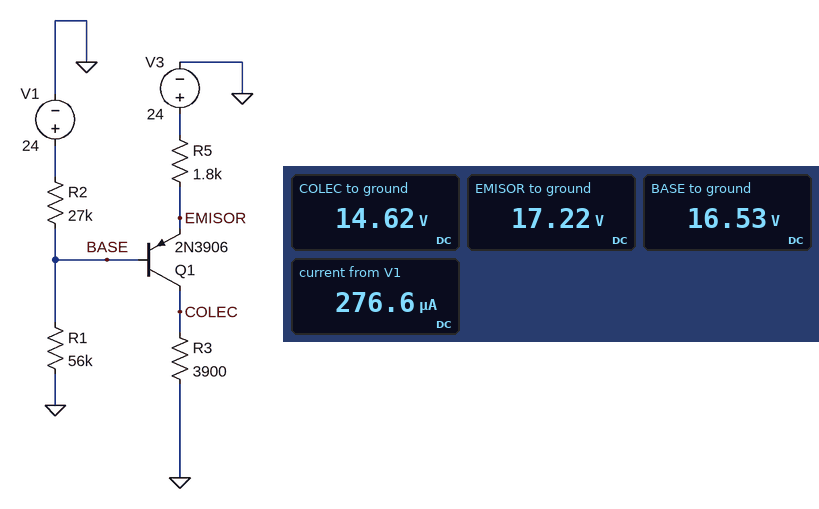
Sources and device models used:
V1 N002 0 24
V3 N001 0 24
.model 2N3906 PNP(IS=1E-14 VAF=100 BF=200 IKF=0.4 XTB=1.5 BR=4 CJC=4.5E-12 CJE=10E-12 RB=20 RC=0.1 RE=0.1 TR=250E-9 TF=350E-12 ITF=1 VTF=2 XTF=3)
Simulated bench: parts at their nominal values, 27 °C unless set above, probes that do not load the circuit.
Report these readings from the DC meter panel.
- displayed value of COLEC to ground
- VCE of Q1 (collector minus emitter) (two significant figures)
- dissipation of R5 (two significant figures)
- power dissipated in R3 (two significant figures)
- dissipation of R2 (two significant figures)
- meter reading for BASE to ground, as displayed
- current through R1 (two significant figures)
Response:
14.62 V
-2.6 V
26 mW
55 mW
2.1 mW
16.53 V
300 µA
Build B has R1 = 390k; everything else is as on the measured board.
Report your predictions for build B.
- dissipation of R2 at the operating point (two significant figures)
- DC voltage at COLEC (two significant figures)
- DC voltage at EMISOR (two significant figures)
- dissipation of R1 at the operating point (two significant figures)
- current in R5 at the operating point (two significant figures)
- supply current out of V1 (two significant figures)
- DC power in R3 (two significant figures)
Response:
84 µW
1.9 V
23 V
1.3 mW
480 µA
56 µA
910 µW
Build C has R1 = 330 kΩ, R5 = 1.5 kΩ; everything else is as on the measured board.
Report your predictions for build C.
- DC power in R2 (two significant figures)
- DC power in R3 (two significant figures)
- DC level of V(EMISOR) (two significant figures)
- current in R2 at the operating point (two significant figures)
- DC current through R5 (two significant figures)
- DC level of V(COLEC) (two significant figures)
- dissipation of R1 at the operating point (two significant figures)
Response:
110 µW
2.1 mW
23 V
64 µA
730 µA
2.8 V
1.5 mW
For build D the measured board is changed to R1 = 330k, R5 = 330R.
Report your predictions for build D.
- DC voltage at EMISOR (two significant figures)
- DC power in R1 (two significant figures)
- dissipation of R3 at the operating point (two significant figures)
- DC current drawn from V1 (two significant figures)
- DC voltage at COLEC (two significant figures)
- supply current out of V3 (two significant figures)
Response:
23 V
1.5 mW
26 mW
57 µA
10 V
2.6 mA
